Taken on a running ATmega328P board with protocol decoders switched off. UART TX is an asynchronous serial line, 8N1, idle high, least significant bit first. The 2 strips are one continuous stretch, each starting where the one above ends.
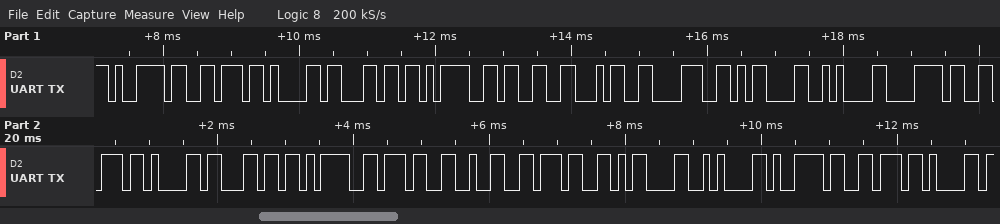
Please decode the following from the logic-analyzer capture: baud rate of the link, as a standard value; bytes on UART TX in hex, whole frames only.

9600 baud
79 76 61 6C 3D 33 34 38 0D 0A 78 76 61 6C 3D 37 32 37 0D 0A 79 76 61
